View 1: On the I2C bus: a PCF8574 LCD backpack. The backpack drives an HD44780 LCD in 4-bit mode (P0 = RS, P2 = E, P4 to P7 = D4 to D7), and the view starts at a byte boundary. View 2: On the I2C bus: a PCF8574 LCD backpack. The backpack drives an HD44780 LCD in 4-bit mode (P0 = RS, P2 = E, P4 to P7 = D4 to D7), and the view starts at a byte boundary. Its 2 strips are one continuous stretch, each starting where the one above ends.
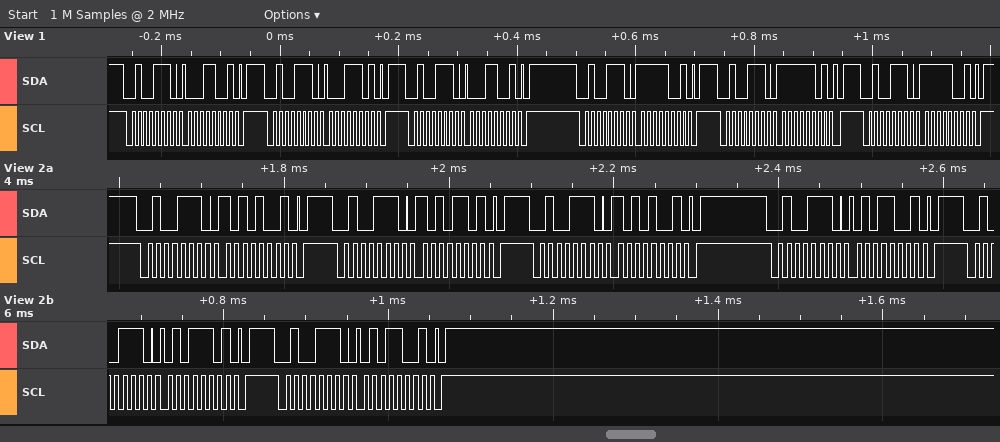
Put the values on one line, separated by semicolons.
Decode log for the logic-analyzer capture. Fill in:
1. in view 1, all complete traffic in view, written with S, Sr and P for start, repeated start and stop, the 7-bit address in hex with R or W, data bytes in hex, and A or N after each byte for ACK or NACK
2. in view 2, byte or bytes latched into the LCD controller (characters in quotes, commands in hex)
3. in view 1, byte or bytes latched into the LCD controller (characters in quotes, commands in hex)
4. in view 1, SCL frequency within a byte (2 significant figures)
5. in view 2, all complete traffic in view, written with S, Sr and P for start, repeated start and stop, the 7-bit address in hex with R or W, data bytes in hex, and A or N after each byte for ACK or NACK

S 27W A 19 A P S 27W A 1D A P S 27W A 19 A P S 27W A F9 A P S 27W A FD A P S 27W A F9 A P; data 0xA5; data 0x1F; 100 kHz; S 27W A A9 A P S 27W A AD A P S 27W A A9 A P S 27W A 59 A P S 27W A 5D A P S 27W A 59 A P
